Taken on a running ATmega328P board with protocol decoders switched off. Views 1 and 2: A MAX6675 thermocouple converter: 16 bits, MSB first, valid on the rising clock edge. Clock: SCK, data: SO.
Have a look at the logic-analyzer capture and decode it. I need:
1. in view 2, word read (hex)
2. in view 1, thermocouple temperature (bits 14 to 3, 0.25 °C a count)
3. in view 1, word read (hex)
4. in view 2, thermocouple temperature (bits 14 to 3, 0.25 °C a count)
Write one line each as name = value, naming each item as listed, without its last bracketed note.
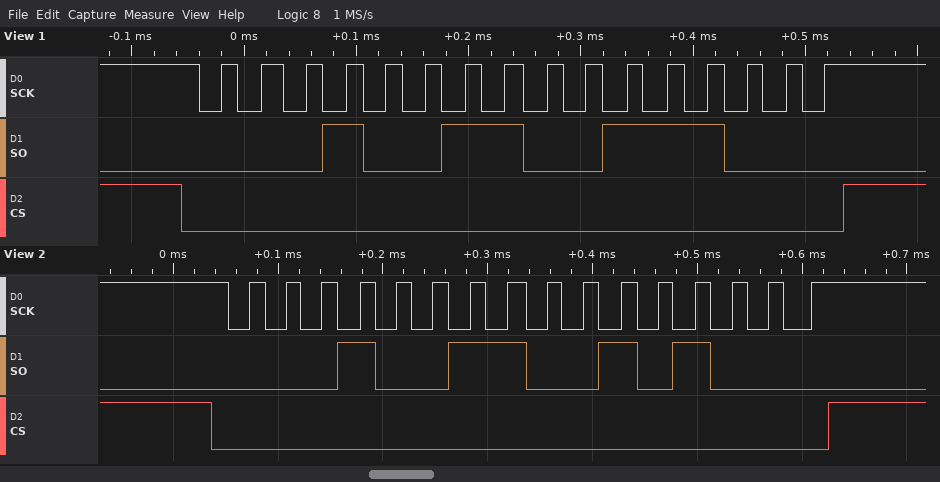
in view 2, word read = 0x1328
in view 1, thermocouple temperature = 153.75 °C
in view 1, word read = 0x1338
in view 2, thermocouple temperature = 153.25 °C
